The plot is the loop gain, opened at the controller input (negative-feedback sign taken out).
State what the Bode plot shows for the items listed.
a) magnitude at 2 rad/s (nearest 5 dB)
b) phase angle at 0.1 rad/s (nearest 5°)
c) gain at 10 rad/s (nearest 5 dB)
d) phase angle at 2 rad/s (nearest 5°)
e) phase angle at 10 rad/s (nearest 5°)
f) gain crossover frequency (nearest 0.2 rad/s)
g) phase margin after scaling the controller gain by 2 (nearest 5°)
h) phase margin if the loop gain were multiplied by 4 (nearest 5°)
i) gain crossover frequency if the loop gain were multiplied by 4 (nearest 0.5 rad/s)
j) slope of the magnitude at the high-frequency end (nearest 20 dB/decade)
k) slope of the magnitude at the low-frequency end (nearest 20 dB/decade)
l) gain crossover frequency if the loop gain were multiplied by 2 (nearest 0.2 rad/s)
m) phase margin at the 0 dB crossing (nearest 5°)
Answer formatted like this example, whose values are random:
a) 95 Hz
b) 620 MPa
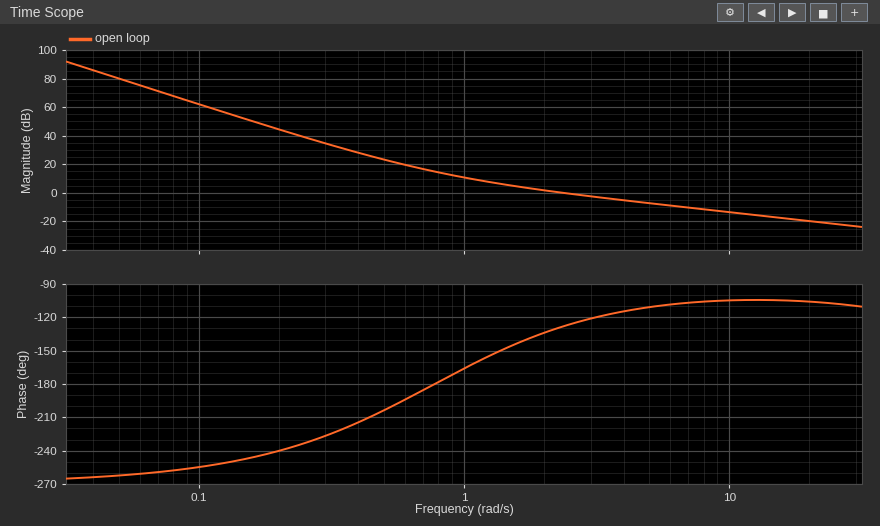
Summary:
a) 0 dB
b) -255°
c) -15 dB
d) -135°
e) -105°
f) 2.4 rad/s
g) 65°
h) 75°
i) 8.5 rad/s
j) -20 dB/decade
k) -60 dB/decade
l) 4.4 rad/s
m) 50°
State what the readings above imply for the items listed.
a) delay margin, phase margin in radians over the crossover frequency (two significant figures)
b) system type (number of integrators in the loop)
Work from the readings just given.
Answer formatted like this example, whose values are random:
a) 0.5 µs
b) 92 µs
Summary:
a) 0.36 s
b) 3
